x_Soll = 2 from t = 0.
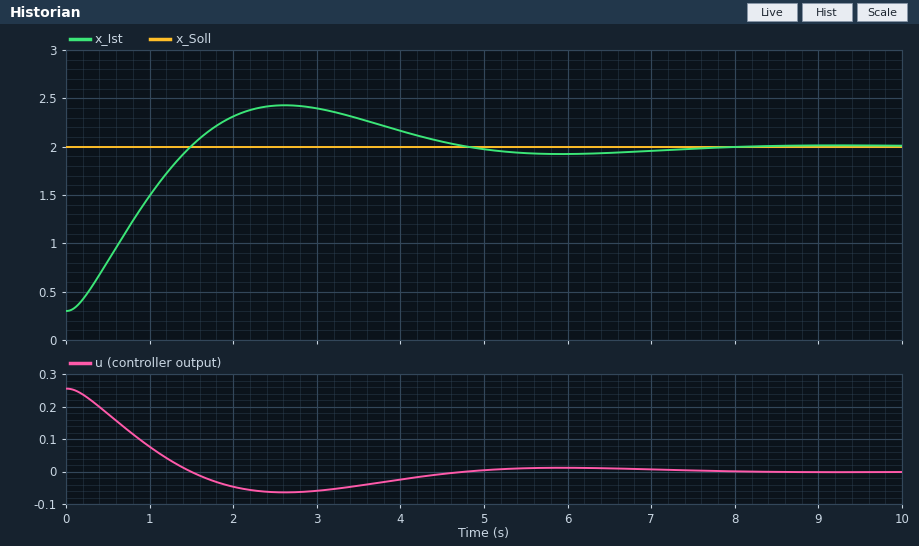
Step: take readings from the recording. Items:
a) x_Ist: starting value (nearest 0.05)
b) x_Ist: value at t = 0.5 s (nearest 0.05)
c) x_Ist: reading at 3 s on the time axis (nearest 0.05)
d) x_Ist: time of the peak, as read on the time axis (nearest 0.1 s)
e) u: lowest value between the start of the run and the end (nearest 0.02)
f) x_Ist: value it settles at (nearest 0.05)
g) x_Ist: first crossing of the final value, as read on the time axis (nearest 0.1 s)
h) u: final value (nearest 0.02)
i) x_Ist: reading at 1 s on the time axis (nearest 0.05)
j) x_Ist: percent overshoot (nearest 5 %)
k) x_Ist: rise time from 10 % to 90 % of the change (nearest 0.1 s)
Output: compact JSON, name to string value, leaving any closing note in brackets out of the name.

{"x_Ist: starting value": "0.30", "x_Ist: value at t = 0.5 s": "0.80", "x_Ist: reading at 3 s on the time axis": "2.40", "x_Ist: time of the peak, as read on the time axis": "2.6 s", "u: lowest value between the start of the run and the end": "-0.06", "x_Ist: value it settles at": "2.00", "x_Ist: first crossing of the final value, as read on the time axis": "1.5 s", "u: final value": "0.00", "x_Ist: reading at 1 s on the time axis": "1.50", "x_Ist: percent overshoot": "25 %", "x_Ist: rise time from 10 % to 90 % of the change": "1.1 s"}
